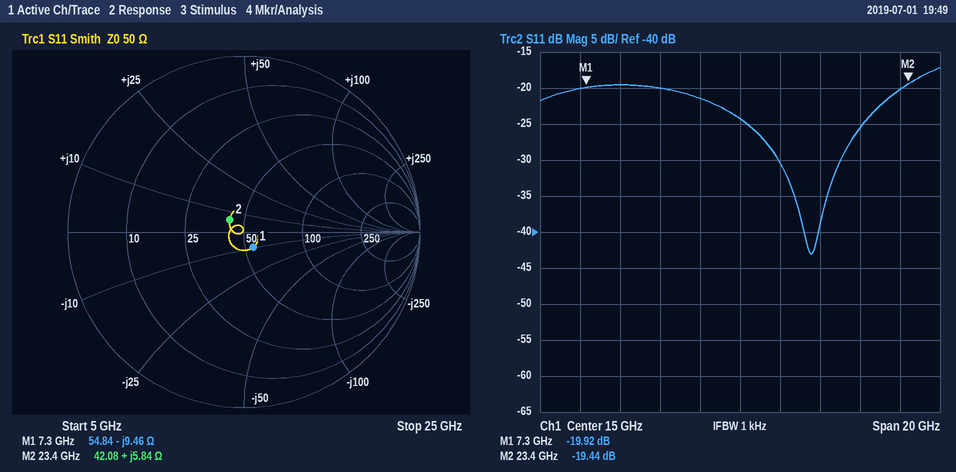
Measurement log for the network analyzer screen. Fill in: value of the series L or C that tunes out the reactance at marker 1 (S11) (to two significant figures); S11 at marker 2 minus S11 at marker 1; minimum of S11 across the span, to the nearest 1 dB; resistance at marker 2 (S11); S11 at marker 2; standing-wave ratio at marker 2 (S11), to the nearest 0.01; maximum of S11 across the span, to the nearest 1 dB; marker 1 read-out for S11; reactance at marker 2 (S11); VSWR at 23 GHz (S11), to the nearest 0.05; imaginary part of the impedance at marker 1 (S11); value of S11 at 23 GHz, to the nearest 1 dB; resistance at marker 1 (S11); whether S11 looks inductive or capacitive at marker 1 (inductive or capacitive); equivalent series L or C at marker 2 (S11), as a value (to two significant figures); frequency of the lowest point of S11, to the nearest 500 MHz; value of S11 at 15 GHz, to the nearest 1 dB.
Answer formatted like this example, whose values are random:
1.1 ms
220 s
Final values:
210 pH
0.48 dB
-43 dB
42.08 Ω
-19.44 dB
1.24
-17 dB
-19.92 dB
+5.84 Ω
1.20
-9.46 Ω
-20 dB
54.84 Ω
capacitive
40 pH
18.5 GHz
-24 dB
